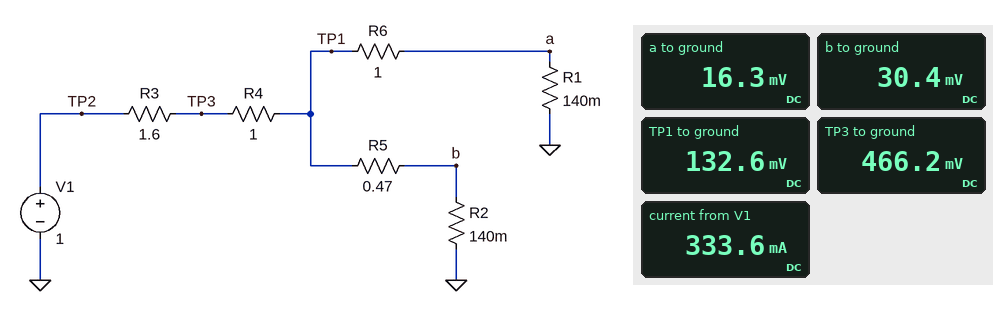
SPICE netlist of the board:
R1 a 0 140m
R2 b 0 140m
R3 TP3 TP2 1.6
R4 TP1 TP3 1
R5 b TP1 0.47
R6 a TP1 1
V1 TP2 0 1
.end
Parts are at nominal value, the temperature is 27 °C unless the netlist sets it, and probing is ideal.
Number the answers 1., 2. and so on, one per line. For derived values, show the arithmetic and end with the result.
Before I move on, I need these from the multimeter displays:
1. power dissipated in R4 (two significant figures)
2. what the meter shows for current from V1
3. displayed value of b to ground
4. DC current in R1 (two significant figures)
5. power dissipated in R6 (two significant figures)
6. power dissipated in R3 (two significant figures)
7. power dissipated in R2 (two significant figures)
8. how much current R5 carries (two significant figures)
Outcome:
1. (466.2 mV - 132.6 mV)^2 / 1 Ω = 110 mW
2. 333.6 mA
3. 30.4 mV
4. (16.3 mV) / 140 mΩ = 120 mA
5. (132.6 mV - 16.3 mV)^2 / 1 Ω = 14 mW
6. (1 V - 466.2 mV)^2 / 1.6 Ω = 180 mW
7. (30.4 mV)^2 / 140 mΩ = 6.6 mW
8. (132.6 mV - 30.4 mV) / 470 mΩ = 220 mA
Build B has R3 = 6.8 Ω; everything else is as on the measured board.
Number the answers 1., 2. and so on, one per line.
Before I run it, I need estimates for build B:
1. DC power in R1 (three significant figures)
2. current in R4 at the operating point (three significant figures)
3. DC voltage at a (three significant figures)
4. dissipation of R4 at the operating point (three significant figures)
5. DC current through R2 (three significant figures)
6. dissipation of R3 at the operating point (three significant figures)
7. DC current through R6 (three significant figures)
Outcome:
1. 253 µW
2. 122 mA
3. 5.95 mV
4. 14.9 mW
5. 79.5 mA
6. 101 mW
7. 42.5 mA
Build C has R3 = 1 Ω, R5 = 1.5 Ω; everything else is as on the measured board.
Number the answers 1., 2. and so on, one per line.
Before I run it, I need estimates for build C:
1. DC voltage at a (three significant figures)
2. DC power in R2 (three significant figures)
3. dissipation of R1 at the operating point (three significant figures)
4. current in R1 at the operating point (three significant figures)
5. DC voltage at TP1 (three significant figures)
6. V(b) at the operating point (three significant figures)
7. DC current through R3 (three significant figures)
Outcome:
1. 30.9 mV
2. 3.30 mW
3. 6.82 mW
4. 221 mA
5. 252 mV
6. 21.5 mV
7. 374 mA
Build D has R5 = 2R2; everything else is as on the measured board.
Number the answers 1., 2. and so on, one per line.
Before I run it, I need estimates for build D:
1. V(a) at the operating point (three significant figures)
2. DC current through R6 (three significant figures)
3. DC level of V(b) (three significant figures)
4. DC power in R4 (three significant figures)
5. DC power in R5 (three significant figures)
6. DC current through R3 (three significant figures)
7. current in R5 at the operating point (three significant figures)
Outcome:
1. 28.0 mV
2. 200 mA
3. 13.6 mV
4. 88.2 mW
5. 20.8 mW
6. 297 mA
7. 97.3 mA
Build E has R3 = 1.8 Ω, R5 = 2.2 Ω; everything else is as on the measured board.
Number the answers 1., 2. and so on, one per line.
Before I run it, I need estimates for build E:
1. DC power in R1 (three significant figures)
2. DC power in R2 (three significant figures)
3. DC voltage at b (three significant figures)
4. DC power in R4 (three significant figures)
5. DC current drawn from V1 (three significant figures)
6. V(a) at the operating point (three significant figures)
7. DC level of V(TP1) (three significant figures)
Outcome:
1. 4.98 mW
2. 1.18 mW
3. 12.9 mV
4. 78.6 mW
5. 280 mA
6. 26.4 mV
7. 215 mV
